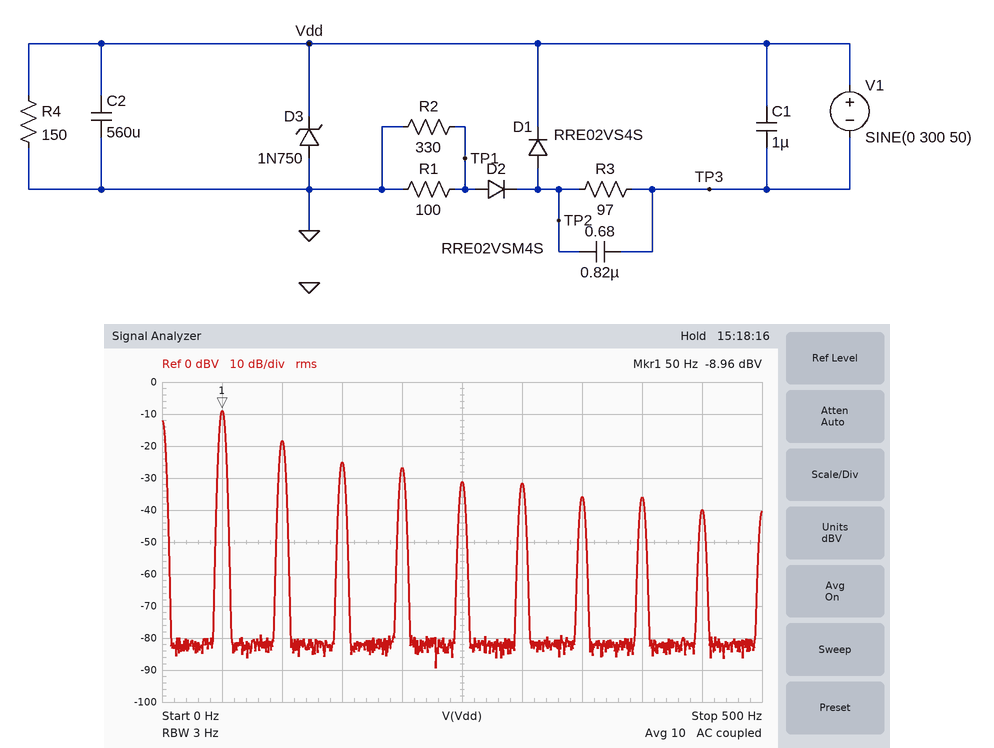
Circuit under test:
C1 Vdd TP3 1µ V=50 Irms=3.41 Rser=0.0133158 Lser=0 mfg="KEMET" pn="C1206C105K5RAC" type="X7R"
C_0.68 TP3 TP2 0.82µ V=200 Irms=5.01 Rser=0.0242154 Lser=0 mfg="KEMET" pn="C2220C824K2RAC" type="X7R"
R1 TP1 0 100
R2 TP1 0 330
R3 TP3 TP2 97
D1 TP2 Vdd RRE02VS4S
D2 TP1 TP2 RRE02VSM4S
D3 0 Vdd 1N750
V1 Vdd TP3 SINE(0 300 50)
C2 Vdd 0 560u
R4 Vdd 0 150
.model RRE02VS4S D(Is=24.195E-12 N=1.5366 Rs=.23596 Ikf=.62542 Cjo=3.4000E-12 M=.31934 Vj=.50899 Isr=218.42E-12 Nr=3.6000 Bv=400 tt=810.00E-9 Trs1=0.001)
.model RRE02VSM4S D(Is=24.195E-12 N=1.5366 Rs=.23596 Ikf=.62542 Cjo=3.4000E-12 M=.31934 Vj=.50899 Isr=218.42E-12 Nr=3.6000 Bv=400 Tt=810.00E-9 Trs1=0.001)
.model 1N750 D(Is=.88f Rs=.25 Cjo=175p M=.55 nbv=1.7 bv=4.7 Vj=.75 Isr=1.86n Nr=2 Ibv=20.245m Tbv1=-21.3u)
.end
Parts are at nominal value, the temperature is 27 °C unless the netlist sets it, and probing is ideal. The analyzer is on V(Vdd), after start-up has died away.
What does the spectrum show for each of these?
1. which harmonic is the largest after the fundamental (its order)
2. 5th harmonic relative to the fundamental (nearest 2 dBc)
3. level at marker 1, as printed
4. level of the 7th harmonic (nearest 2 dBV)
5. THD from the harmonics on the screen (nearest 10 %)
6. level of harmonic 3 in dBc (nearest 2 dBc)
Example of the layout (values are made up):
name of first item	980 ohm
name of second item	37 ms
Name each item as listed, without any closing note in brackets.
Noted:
which harmonic is the largest after the fundamental	2
5th harmonic relative to the fundamental	-22 dBc
level at marker 1, as printed	-8.96 dBV
level of the 7th harmonic	-36 dBV
THD from the harmonics on the screen	40 %
level of harmonic 3 in dBc	-16 dBc
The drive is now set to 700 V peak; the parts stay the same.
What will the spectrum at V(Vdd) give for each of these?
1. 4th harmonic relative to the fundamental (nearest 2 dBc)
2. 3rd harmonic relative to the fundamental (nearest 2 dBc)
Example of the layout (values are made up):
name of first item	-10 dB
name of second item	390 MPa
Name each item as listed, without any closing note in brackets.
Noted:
4th harmonic relative to the fundamental	-20 dBc
3rd harmonic relative to the fundamental	-20 dBc
